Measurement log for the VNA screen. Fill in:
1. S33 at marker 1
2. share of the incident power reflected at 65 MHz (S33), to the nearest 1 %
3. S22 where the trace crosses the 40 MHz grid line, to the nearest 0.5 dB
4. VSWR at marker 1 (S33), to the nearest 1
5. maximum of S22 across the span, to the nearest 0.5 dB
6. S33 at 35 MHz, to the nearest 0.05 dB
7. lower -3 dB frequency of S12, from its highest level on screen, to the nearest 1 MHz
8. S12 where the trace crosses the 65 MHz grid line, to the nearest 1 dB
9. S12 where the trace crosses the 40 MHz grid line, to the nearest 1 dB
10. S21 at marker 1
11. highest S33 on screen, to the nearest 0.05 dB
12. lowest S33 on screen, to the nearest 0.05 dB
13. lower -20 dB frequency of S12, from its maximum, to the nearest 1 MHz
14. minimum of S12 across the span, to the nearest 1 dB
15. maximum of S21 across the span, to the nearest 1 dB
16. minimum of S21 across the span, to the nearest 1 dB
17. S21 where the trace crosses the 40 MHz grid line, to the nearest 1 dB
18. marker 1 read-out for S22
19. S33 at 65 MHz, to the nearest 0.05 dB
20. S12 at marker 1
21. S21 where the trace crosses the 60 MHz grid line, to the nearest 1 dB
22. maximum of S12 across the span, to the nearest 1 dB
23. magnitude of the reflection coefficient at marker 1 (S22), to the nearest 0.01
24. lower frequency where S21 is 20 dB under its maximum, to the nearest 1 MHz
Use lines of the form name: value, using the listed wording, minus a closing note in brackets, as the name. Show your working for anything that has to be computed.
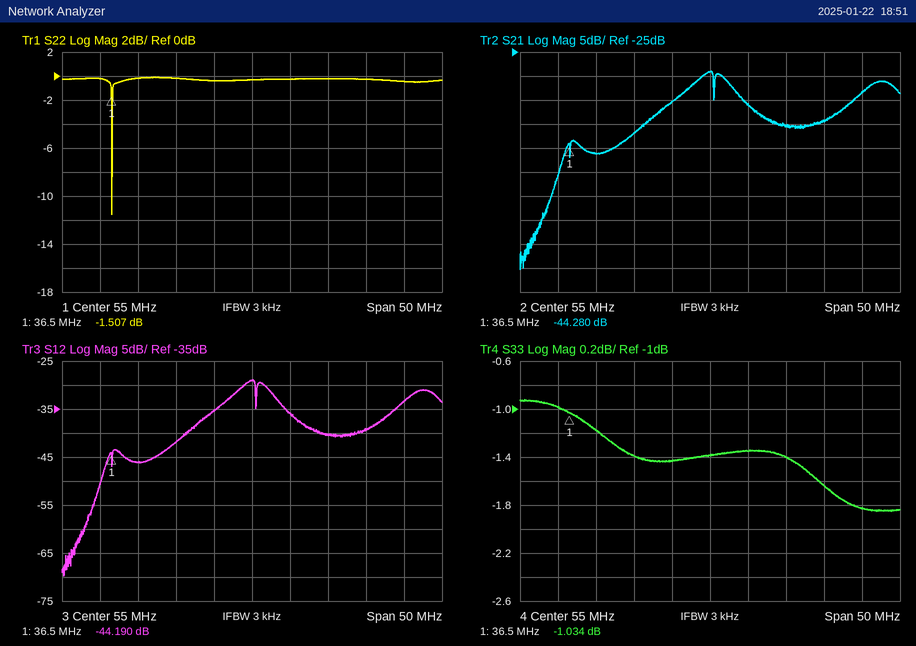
S33 at marker 1: -1.034 dB
share of the incident power reflected at 65 MHz (S33), to the nearest 1 %: 10^(-1.4/10) ≈ 72 %
S22 where the trace crosses the 40 MHz grid line, to the nearest 0.5 dB: 0.0 dB
VSWR at marker 1 (S33), to the nearest 1: (1 + 0.8878)/(1 − 0.8878) ≈ 17
maximum of S22 across the span, to the nearest 0.5 dB: 0.0 dB
S33 at 35 MHz, to the nearest 0.05 dB: -1.00 dB
lower -3 dB frequency of S12, from its highest level on screen, to the nearest 1 MHz: 53 MHz
S12 where the trace crosses the 65 MHz grid line, to the nearest 1 dB: -40 dB
S12 where the trace crosses the 40 MHz grid line, to the nearest 1 dB: -46 dB
S21 at marker 1: -44.280 dB
highest S33 on screen, to the nearest 0.05 dB: -0.90 dB
lowest S33 on screen, to the nearest 0.05 dB: -1.85 dB
lower -20 dB frequency of S12, from its maximum, to the nearest 1 MHz: 35 MHz
minimum of S12 across the span, to the nearest 1 dB: -70 dB
maximum of S21 across the span, to the nearest 1 dB: -29 dB
minimum of S21 across the span, to the nearest 1 dB: -70 dB
S21 where the trace crosses the 40 MHz grid line, to the nearest 1 dB: -46 dB
marker 1 read-out for S22: -1.507 dB
S33 at 65 MHz, to the nearest 0.05 dB: -1.40 dB
S12 at marker 1: -44.190 dB
S21 where the trace crosses the 60 MHz grid line, to the nearest 1 dB: -36 dB
maximum of S12 across the span, to the nearest 1 dB: -29 dB
magnitude of the reflection coefficient at marker 1 (S22), to the nearest 0.01: 10^(-1.507/20) ≈ 0.84
lower frequency where S21 is 20 dB under its maximum, to the nearest 1 MHz: 35 MHz
